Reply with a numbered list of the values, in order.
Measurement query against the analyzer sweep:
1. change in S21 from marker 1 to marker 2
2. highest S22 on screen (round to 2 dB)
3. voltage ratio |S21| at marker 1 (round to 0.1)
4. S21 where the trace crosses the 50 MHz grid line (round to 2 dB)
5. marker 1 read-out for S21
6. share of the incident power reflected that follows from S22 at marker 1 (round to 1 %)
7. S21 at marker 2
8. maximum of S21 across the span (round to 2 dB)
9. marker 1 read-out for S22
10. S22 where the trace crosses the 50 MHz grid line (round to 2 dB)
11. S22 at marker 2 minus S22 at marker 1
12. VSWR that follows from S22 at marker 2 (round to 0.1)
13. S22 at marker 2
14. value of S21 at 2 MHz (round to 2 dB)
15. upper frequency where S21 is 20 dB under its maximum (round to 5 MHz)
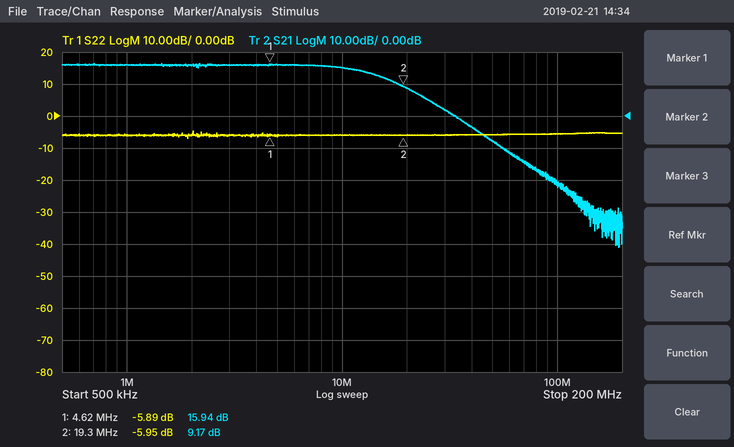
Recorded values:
1. -6.77 dB
2. -4 dB
3. 6.3
4. -8 dB
5. 15.94 dB
6. 26 %
7. 9.17 dB
8. 16 dB
9. -5.89 dB
10. -6 dB
11. -0.06 dB
12. 3.0
13. -5.95 dB
14. 16 dB
15. 40 MHz
